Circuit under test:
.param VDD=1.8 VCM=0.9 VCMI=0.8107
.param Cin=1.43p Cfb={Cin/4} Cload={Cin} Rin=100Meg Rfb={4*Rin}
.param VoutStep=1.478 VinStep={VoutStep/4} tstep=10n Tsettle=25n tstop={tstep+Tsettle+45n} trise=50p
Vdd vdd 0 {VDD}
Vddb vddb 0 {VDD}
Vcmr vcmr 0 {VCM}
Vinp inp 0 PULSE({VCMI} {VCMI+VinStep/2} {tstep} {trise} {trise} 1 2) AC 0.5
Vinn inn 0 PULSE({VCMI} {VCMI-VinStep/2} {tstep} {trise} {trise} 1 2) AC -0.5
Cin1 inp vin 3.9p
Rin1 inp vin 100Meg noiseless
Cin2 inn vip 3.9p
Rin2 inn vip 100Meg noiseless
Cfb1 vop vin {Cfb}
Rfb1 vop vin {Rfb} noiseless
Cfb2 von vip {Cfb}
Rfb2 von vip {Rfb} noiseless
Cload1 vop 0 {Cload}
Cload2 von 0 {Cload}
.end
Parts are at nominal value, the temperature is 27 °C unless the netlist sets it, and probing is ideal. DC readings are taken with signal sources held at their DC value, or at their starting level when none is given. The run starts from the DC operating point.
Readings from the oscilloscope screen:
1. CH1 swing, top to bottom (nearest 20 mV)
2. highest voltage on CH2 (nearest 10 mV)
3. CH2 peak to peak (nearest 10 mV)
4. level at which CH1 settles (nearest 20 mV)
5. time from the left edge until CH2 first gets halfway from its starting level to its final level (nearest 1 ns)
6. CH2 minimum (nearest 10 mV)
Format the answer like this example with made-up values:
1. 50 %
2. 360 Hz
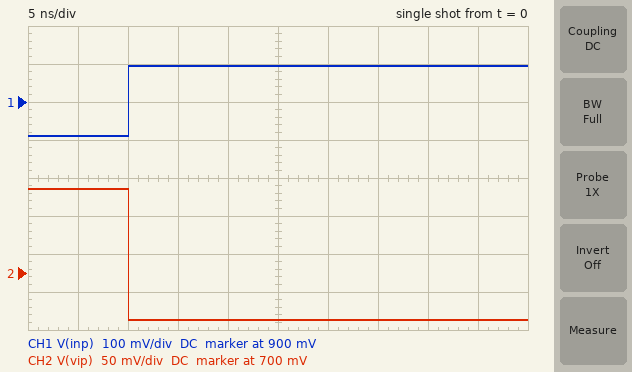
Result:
1. 180 mV
2. 810 mV
3. 170 mV
4. 1.00 V
5. 10 ns
6. 640 mV
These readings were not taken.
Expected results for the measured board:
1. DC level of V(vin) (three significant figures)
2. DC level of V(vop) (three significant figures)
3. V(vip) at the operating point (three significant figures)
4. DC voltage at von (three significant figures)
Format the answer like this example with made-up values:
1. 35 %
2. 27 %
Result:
1. 811 mV
2. 811 mV
3. 811 mV
4. 811 mV
